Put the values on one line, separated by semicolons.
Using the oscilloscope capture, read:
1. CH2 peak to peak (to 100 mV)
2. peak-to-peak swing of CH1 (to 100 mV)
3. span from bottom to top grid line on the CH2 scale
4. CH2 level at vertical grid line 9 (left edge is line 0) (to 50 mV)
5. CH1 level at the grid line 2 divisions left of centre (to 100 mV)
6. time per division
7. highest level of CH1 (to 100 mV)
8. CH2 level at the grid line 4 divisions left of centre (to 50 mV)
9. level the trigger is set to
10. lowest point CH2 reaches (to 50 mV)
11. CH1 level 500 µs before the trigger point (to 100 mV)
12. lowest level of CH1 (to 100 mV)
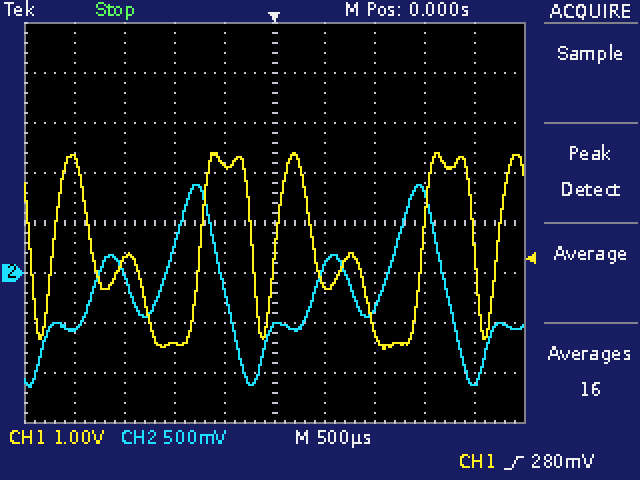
2.00 V; 3.9 V; 4 V; -1.10 V; -1.4 V; 500 µs; 2.4 V; -550 mV; 280 mV; -1.15 V; 2.2 V; -1.5 V
